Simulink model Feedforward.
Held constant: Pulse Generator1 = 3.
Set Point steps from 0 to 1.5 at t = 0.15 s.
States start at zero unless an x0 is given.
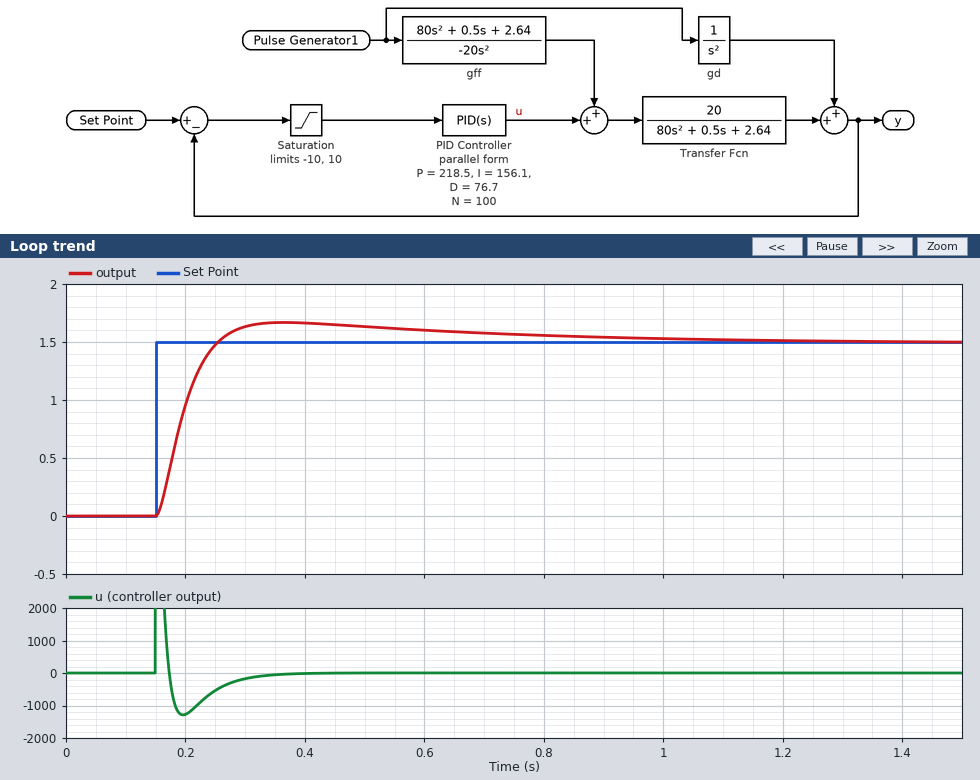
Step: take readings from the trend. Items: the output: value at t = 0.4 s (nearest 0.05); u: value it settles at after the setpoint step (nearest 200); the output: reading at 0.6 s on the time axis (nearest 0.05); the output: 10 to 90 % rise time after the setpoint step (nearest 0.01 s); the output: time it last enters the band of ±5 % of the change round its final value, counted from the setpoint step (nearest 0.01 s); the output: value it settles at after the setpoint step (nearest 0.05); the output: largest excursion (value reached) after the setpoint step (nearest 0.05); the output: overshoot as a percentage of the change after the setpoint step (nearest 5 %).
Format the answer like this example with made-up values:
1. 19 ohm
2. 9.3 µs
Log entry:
1. 1.65
2. 0
3. 1.60
4. 0.07 s
5. 0.56 s
6. 1.50
7. 1.65
8. 10 %
